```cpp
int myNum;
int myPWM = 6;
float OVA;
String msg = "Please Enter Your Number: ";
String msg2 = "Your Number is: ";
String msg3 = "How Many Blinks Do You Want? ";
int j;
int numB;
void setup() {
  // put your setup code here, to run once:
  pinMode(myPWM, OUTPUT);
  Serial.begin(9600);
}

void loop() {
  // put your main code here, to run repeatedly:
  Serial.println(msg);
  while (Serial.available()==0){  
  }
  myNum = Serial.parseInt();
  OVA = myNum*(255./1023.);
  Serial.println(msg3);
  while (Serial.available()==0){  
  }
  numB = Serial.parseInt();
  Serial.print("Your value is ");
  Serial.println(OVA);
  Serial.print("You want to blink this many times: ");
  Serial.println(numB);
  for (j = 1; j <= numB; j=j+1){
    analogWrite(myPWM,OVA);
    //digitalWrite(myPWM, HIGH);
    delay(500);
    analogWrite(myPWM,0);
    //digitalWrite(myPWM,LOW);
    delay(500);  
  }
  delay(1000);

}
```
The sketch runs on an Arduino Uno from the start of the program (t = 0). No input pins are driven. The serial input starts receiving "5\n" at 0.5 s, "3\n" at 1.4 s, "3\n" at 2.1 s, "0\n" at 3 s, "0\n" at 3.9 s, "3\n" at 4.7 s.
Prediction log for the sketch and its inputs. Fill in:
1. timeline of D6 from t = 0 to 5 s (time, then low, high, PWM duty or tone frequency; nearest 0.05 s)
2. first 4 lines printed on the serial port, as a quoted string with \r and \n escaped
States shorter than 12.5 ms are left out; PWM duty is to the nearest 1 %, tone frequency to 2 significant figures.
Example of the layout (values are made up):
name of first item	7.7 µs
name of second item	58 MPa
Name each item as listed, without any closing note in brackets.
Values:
timeline of D6 from t = 0 to 5 s	0 s low; 1.4 s PWM 1 %; 1.9 s low; 2.4 s PWM 1 %; 2.9 s low; 3.4 s PWM 1 %; 3.9 s low
first 4 lines printed on the serial port, as a quoted string with \r and \n escaped	"Please Enter Your Number: \r\nHow Many Blinks Do You Want? \r\nYour value is 1.25\r\nYou want to blink this many times: 3\r\n"
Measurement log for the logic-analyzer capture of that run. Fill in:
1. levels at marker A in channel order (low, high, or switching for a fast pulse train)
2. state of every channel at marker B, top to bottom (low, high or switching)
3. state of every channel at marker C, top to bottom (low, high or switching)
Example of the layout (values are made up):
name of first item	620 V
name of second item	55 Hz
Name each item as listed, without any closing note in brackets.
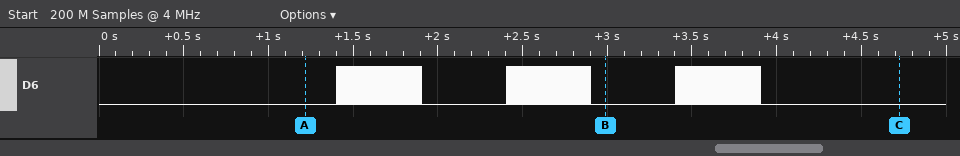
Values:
levels at marker A in channel order	D6 low
state of every channel at marker B, top to bottom	D6 low
state of every channel at marker C, top to bottom	D6 low
